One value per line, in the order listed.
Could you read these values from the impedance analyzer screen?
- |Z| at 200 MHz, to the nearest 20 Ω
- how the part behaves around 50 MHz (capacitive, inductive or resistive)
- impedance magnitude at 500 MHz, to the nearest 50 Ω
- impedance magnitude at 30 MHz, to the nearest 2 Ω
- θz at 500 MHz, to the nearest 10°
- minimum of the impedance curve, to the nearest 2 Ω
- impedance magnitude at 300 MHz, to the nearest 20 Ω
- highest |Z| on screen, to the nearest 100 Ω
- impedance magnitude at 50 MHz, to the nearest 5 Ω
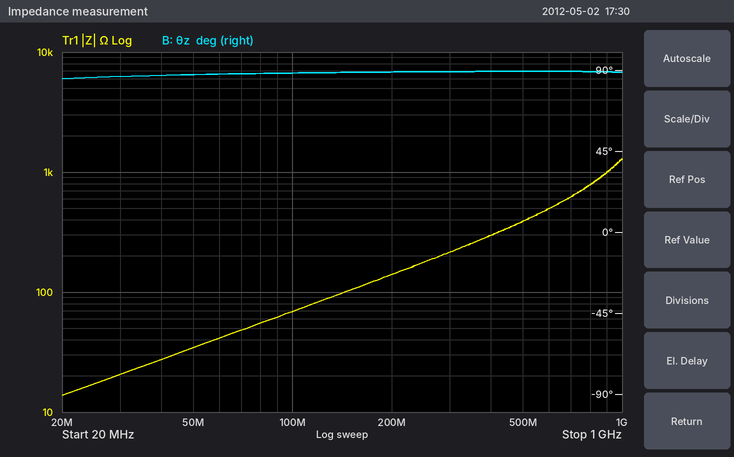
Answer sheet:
140 Ω
inductive
400 Ω
20 Ω
90°
14 Ω
220 Ω
1.3 kΩ
35 Ω
